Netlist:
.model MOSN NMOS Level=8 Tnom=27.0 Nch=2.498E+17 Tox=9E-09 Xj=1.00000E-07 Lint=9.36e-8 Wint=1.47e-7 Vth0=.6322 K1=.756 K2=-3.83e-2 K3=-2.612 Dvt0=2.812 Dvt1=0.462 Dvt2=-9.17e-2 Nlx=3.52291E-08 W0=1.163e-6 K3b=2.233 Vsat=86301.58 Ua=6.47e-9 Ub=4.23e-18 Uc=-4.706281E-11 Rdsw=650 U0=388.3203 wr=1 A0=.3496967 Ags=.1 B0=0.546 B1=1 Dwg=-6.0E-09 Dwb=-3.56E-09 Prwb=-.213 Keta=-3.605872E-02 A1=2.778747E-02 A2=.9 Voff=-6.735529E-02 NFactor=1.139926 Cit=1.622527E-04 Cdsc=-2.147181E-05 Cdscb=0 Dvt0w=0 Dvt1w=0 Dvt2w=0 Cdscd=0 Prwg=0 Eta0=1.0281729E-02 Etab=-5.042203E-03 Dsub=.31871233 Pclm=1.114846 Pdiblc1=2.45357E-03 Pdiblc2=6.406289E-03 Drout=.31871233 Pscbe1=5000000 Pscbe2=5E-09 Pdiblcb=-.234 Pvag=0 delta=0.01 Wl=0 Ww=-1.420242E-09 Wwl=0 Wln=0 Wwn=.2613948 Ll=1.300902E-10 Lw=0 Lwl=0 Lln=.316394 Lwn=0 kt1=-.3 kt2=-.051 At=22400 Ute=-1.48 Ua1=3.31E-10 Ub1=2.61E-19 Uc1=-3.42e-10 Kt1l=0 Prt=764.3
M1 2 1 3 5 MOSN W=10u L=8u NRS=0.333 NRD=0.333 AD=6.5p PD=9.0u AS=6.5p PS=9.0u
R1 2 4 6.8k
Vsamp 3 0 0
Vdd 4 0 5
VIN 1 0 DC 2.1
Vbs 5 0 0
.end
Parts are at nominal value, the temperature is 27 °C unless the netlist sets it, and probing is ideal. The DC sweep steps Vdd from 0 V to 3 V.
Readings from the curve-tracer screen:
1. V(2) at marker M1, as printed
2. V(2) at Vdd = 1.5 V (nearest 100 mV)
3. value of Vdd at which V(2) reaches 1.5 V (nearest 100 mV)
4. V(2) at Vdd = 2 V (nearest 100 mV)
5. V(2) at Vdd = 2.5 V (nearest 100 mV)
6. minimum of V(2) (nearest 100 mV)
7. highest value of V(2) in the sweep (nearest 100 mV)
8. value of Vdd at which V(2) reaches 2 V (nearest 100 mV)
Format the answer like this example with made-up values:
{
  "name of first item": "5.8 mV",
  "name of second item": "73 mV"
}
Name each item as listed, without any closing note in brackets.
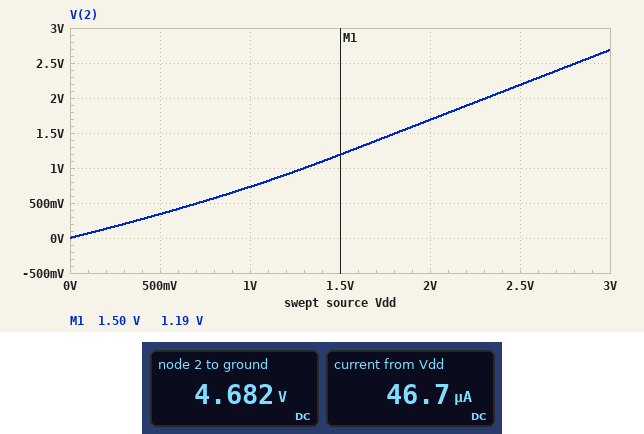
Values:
{
  "V(2) at marker M1, as printed": "1.19 V",
  "V(2) at Vdd = 1.5 V": "1.2 V",
  "value of Vdd at which V(2) reaches 1.5 V": "1.8 V",
  "V(2) at Vdd = 2 V": "1.7 V",
  "V(2) at Vdd = 2.5 V": "2.2 V",
  "minimum of V(2)": "0 V",
  "highest value of V(2) in the sweep": "2.7 V",
  "value of Vdd at which V(2) reaches 2 V": "2.3 V"
}
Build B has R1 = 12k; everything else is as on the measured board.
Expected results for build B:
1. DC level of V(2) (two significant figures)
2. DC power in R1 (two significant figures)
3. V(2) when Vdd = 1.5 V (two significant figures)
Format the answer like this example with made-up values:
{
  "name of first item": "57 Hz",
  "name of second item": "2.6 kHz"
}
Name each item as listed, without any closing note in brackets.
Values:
{
  "DC level of V(2)": "4.4 V",
  "DC power in R1": "26 µW",
  "V(2) when Vdd = 1.5 V": "970 mV"
}
